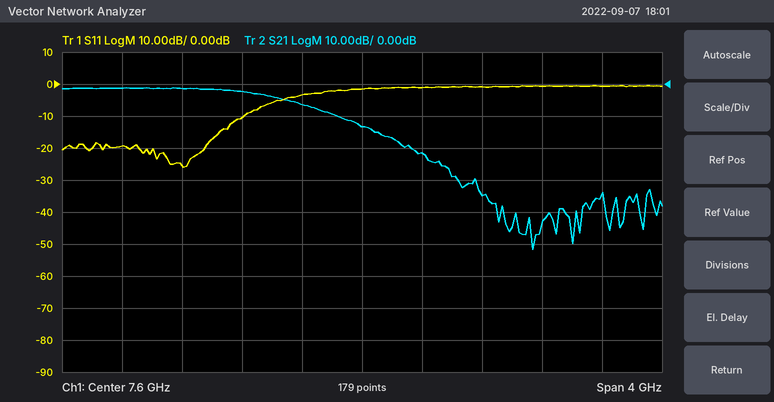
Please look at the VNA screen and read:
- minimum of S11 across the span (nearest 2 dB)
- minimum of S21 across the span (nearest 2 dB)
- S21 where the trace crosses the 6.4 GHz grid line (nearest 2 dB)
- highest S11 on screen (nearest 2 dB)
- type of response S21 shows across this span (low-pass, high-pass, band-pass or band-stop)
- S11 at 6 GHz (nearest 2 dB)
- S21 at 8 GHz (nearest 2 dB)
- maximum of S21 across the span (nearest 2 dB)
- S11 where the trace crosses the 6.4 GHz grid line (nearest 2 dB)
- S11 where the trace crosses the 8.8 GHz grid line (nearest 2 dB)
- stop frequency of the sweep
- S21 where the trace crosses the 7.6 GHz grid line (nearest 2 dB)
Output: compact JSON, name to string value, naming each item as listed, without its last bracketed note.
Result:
{"minimum of S11 across the span": "-26 dB", "minimum of S21 across the span": "-52 dB", "S21 where the trace crosses the 6.4 GHz grid line": "-2 dB", "highest S11 on screen": "0 dB", "type of response S21 shows across this span": "low-pass", "S11 at 6 GHz": "-20 dB", "S21 at 8 GHz": "-22 dB", "maximum of S21 across the span": "-2 dB", "S11 where the trace crosses the 6.4 GHz grid line": "-26 dB", "S11 where the trace crosses the 8.8 GHz grid line": "0 dB", "stop frequency of the sweep": "9.6 GHz", "S21 where the trace crosses the 7.6 GHz grid line": "-14 dB"}
